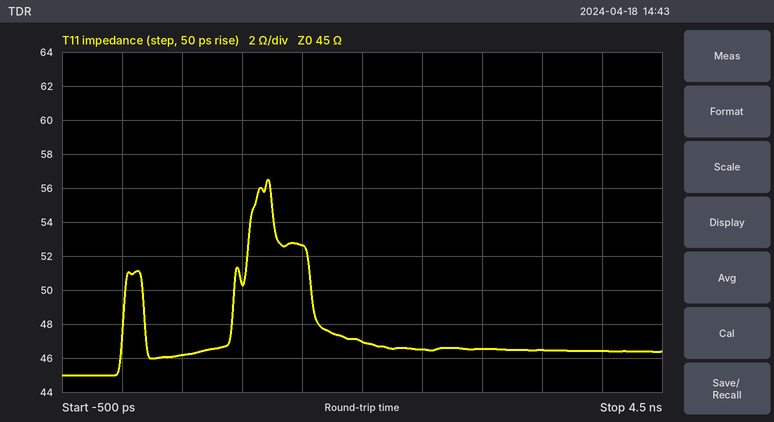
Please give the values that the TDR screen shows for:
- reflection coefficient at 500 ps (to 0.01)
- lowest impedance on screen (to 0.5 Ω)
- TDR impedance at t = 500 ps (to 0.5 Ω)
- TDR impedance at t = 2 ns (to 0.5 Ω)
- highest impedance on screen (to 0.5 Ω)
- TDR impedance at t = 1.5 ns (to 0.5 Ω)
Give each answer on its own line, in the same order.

+0.01
45.0 Ω
46.0 Ω
47.0 Ω
56.5 Ω
52.5 Ω
